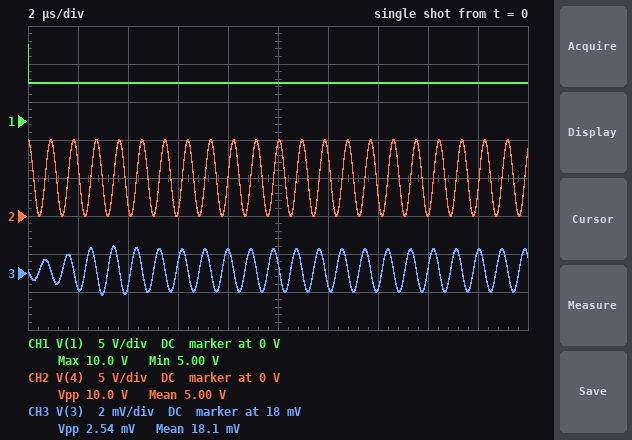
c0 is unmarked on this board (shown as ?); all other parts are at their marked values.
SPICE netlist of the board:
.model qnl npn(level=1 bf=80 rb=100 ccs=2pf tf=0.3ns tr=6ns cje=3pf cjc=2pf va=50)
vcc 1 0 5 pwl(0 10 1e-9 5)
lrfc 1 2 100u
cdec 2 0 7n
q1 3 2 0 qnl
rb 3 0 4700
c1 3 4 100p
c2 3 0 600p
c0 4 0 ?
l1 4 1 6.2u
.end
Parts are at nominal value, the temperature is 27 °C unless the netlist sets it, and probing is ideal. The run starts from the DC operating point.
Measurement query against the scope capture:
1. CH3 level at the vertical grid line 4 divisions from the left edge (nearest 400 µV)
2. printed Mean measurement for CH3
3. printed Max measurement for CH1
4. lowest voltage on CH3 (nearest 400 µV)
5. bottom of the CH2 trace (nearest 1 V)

19.2 mV
18.1 mV
10.0 V
16.8 mV
0 V
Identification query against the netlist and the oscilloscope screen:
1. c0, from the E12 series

3.3 nF
